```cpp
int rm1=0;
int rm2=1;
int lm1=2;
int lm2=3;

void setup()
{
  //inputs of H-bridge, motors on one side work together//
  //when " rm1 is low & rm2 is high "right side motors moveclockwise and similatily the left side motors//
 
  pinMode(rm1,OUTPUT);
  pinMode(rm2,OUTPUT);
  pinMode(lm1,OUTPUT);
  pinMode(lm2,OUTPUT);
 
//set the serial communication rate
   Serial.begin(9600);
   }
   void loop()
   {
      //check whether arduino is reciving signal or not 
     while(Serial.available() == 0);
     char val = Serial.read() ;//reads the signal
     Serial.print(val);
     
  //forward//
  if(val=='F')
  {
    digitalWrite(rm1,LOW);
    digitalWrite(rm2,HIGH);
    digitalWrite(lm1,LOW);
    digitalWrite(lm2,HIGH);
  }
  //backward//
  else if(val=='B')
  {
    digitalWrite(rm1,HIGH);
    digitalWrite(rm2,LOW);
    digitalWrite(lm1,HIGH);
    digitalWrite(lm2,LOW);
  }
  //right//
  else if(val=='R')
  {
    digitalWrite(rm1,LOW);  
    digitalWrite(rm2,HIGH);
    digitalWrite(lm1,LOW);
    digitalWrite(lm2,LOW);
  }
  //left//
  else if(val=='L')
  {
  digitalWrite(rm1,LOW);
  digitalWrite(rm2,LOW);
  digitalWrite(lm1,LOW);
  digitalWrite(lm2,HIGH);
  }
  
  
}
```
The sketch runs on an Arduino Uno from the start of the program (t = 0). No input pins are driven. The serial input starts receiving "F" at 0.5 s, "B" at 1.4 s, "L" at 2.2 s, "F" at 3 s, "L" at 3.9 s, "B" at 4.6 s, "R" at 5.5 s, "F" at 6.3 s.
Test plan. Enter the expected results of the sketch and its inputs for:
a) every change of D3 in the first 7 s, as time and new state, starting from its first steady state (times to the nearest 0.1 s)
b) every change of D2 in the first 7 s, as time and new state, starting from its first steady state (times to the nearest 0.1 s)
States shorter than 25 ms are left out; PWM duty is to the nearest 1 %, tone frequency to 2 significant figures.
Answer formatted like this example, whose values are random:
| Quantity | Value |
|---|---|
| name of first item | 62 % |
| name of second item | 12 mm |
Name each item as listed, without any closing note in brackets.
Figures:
| Quantity | Value |
|---|---|
| every change of D3 in the first 7 s, as time and new state, starting from its first steady state | 0 s low; 0.5 s high; 1.4 s low; 2.2 s high; 4.6 s low; 6.3 s high |
| every change of D2 in the first 7 s, as time and new state, starting from its first steady state | 0 s low; 1.4 s high; 2.2 s low; 4.6 s high; 5.5 s low |
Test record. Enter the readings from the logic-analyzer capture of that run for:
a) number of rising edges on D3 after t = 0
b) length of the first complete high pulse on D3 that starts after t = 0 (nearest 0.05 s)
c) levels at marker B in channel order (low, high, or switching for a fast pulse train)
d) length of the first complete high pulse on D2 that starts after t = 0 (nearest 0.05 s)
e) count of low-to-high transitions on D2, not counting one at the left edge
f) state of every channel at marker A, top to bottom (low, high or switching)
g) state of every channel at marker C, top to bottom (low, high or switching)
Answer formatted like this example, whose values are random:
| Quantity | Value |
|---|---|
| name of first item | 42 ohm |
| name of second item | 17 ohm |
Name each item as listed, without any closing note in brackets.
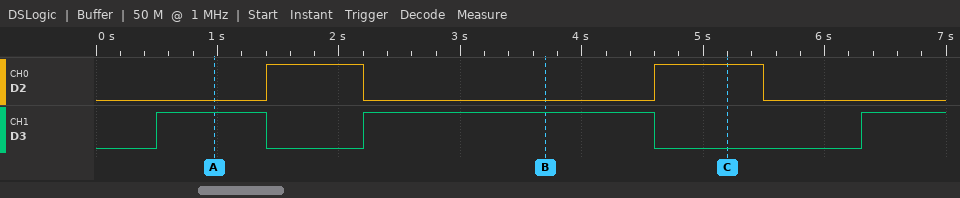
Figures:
| Quantity | Value |
|---|---|
| number of rising edges on D3 after t = 0 | 3 |
| length of the first complete high pulse on D3 that starts after t = 0 | 0.90 s |
| levels at marker B in channel order | D2 low, D3 high |
| length of the first complete high pulse on D2 that starts after t = 0 | 0.80 s |
| count of low-to-high transitions on D2, not counting one at the left edge | 2 |
| state of every channel at marker A, top to bottom | D2 low, D3 high |
| state of every channel at marker C, top to bottom | D2 high, D3 low |
